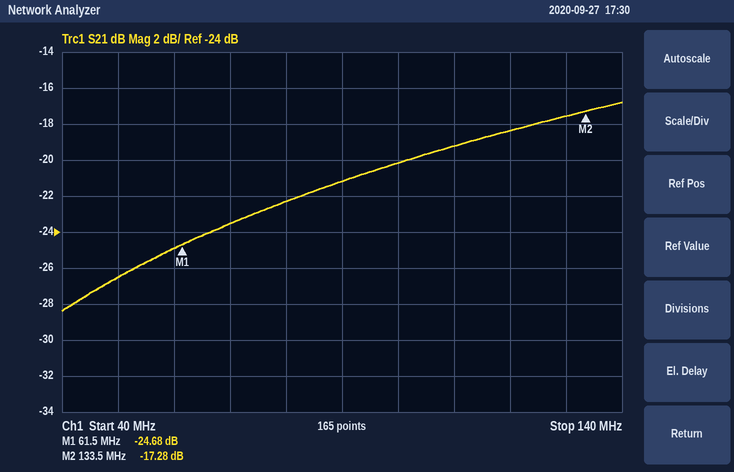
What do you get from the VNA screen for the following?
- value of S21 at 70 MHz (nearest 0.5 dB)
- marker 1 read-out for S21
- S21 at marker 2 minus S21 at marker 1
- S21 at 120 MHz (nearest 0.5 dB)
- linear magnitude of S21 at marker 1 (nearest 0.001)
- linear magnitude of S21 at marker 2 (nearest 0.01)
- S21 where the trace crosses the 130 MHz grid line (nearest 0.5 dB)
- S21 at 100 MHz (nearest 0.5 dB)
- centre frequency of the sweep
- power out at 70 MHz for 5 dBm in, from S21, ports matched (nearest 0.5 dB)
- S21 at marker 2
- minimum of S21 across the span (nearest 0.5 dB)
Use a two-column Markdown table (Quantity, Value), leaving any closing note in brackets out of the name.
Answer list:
| Quantity | Value |
|---|---|
| value of S21 at 70 MHz | -23.5 dB |
| marker 1 read-out for S21 | -24.68 dB |
| S21 at marker 2 minus S21 at marker 1 | 7.40 dB |
| S21 at 120 MHz | -18.5 dB |
| linear magnitude of S21 at marker 1 | 0.058 |
| linear magnitude of S21 at marker 2 | 0.14 |
| S21 where the trace crosses the 130 MHz grid line | -17.5 dB |
| S21 at 100 MHz | -20.0 dB |
| centre frequency of the sweep | 90 MHz |
| power out at 70 MHz for 5 dBm in, from S21, ports matched | -18.5 dBm |
| S21 at marker 2 | -17.28 dB |
| minimum of S21 across the span | -28.5 dB |
